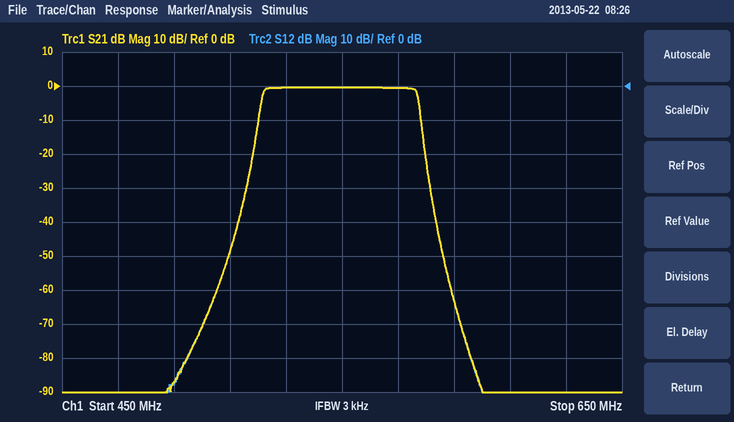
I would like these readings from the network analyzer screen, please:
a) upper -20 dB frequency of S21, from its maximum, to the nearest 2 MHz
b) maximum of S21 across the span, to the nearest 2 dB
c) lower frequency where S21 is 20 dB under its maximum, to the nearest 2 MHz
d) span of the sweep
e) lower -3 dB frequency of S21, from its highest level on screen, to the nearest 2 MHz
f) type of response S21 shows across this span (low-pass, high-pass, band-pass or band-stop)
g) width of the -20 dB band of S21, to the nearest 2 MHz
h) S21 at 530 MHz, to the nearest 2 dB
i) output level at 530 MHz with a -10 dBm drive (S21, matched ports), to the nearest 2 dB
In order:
580 MHz
0 dB
518 MHz
200 MHz
522 MHz
band-pass
62 MHz
0 dB
-10 dBm
